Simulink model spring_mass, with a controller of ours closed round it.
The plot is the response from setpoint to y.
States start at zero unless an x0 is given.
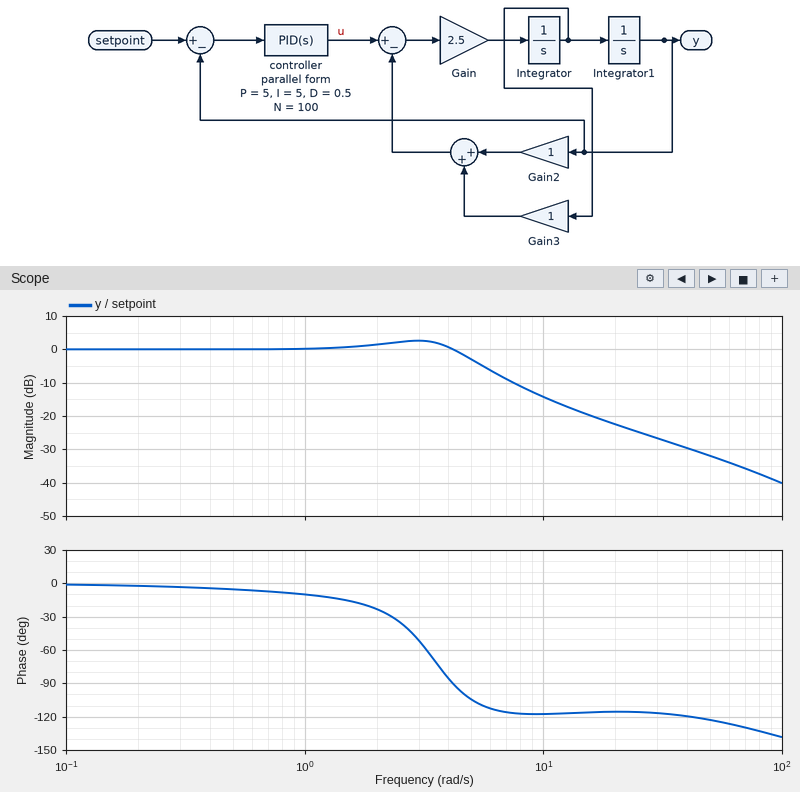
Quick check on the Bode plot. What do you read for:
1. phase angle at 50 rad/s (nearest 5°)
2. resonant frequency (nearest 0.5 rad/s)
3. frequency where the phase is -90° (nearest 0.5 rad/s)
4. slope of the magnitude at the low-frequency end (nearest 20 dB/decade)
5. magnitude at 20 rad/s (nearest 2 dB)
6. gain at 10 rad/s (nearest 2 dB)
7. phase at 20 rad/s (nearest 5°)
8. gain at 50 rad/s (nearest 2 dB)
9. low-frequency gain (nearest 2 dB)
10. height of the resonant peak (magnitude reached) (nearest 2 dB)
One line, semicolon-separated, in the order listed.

-125°; 3.0 rad/s; 4.0 rad/s; 0 dB/decade; -22 dB; -14 dB; -115°; -32 dB; 0 dB; 2 dB
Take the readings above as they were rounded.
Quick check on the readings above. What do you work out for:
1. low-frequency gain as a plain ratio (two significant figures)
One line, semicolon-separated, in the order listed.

1.0
